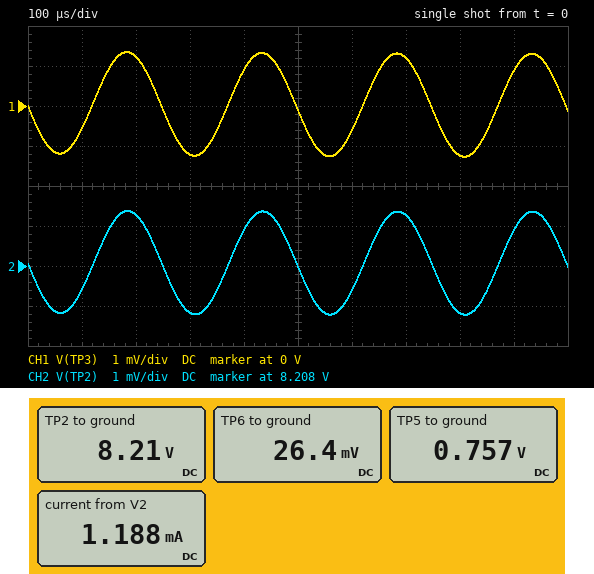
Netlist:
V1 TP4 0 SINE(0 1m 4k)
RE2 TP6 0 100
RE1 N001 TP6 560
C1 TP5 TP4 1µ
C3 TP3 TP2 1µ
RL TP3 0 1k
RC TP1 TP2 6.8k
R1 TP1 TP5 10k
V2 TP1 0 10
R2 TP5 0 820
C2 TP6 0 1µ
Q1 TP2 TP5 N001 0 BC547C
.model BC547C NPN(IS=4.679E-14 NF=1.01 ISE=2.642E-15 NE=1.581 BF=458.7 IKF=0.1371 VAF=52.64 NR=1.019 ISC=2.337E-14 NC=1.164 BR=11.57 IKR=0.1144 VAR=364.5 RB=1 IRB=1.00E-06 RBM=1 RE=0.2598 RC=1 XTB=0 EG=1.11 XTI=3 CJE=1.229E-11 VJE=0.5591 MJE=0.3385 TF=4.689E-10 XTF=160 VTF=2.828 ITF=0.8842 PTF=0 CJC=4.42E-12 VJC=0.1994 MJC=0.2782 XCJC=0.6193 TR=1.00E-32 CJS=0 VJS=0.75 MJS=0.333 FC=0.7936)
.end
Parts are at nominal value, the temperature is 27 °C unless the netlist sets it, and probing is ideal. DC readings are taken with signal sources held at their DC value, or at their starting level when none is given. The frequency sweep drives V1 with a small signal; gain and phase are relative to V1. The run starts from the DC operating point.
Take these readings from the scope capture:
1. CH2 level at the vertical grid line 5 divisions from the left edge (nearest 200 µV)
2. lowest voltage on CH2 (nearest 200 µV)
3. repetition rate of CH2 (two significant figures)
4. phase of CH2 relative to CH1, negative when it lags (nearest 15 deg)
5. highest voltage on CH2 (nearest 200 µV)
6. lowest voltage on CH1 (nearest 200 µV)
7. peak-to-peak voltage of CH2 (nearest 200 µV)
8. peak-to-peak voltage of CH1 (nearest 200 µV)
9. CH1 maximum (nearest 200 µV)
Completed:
8.2080 V
8.2068 V
4.0 kHz
0 deg
8.2094 V
-1.2 mV
2.6 mV
2.6 mV
1.4 mV
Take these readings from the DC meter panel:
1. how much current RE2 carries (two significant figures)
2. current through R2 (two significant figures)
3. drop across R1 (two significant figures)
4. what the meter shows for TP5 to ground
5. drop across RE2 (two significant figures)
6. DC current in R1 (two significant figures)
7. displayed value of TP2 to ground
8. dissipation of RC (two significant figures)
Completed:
260 µA
920 µA
9.2 V
0.757 V
26 mV
920 µA
8.21 V
470 µW
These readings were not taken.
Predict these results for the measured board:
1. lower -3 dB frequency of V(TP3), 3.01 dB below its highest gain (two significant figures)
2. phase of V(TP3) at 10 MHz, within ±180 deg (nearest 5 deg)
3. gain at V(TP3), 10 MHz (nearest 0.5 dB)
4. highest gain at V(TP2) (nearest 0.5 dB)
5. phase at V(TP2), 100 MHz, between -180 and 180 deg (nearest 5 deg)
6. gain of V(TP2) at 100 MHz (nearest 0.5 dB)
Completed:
290 Hz
160 deg
2.5 dB
2.5 dB
60 deg
1.0 dB
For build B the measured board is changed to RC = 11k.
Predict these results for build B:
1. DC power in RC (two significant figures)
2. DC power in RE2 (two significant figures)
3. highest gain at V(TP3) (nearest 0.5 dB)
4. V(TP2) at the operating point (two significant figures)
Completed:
760 µW
6.9 µW
3.0 dB
7.1 V
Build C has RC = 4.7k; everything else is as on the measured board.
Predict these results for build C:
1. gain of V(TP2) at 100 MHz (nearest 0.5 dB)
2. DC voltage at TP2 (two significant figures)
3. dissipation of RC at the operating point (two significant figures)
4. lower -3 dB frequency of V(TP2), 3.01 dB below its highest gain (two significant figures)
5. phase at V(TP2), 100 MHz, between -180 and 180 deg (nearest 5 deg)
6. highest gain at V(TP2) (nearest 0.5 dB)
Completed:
0.5 dB
8.8 V
330 µW
130 Hz
65 deg
2.0 dB
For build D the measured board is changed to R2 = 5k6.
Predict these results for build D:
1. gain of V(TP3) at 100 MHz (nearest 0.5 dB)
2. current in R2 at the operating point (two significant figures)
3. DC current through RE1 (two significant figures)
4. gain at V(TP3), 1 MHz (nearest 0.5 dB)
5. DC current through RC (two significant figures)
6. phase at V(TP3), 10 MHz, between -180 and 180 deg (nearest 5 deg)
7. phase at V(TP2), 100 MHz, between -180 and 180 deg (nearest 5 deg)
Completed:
0 dB
330 µA
1.8 mA
-1.5 dB
1.3 mA
5 deg
0 deg
